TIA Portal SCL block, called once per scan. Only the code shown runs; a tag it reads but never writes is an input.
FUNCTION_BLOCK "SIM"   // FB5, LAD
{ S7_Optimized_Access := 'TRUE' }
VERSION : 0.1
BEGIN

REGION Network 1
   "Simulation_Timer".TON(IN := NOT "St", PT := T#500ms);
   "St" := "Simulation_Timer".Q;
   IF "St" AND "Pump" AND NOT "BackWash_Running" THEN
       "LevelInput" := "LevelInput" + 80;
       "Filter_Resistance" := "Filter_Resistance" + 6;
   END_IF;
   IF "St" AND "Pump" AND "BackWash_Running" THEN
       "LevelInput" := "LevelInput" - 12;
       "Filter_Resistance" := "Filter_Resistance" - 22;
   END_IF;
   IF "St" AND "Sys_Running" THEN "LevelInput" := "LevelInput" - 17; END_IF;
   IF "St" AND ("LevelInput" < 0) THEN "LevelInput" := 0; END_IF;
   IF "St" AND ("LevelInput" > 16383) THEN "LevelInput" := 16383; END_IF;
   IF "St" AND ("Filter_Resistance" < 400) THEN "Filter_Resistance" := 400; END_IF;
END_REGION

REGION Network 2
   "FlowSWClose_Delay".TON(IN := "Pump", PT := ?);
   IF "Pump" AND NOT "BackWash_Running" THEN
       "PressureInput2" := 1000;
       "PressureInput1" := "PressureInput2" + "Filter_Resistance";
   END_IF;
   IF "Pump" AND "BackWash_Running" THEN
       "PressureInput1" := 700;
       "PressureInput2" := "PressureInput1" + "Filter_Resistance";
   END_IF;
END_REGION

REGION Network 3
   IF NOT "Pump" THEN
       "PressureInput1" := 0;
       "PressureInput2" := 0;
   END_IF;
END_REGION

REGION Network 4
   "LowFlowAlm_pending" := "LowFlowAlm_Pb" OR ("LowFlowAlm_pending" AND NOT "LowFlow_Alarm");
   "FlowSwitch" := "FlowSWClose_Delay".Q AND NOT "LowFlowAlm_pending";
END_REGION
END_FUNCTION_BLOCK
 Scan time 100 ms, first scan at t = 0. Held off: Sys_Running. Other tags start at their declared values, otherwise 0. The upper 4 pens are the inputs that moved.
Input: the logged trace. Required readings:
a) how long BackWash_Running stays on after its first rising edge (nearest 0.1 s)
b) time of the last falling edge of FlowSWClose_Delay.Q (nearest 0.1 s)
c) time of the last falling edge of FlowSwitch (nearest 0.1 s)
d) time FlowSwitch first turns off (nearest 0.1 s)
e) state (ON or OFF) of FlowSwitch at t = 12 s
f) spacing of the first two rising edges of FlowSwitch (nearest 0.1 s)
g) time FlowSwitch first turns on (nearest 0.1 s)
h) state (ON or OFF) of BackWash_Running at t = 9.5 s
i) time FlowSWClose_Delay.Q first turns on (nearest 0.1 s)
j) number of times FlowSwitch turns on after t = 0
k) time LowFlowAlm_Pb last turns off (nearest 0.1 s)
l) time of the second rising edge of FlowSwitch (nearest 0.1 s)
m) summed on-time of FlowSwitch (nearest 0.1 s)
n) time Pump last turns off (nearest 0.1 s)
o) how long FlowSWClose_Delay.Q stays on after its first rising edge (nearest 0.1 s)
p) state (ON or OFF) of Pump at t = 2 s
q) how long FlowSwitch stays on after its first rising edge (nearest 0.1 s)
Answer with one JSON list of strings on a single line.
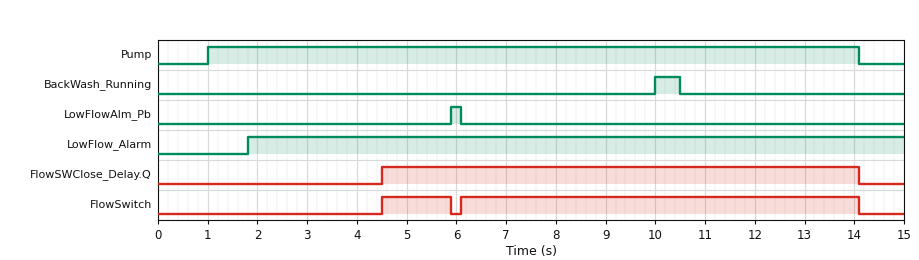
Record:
["0.5 s", "14.1 s", "14.1 s", "5.9 s", "ON", "1.6 s", "4.5 s", "OFF", "4.5 s", "2", "6.1 s", "6.1 s", "9.4 s", "14.1 s", "9.6 s", "ON", "1.4 s"]
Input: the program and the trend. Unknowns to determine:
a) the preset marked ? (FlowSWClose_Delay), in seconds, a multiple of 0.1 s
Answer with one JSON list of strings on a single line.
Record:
["3.5 s"]
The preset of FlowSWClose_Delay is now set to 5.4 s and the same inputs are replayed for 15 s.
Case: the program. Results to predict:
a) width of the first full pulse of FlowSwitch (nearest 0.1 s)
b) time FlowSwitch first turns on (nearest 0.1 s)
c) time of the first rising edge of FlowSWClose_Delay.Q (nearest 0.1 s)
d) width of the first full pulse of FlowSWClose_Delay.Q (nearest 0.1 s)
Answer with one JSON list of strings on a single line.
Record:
["7.7 s", "6.4 s", "6.4 s", "7.7 s"]
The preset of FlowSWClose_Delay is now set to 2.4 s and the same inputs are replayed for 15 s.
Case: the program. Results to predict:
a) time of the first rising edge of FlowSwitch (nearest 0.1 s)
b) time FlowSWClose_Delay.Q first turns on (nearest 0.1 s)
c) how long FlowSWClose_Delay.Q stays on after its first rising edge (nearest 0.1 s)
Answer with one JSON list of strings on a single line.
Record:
["3.4 s", "3.4 s", "10.7 s"]
